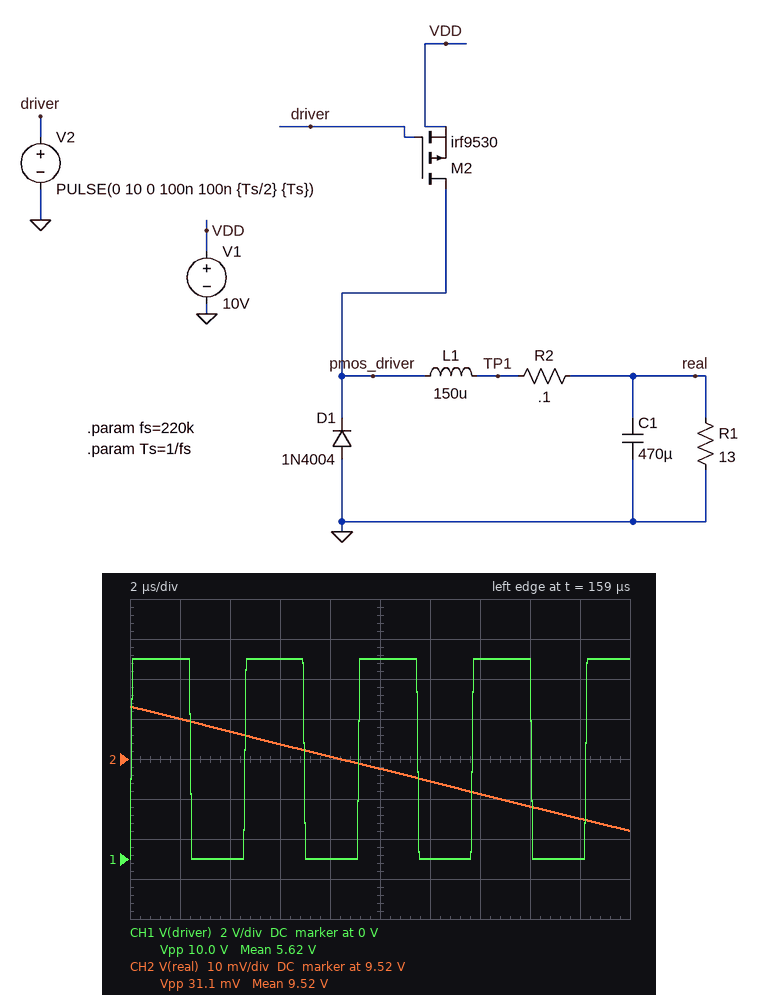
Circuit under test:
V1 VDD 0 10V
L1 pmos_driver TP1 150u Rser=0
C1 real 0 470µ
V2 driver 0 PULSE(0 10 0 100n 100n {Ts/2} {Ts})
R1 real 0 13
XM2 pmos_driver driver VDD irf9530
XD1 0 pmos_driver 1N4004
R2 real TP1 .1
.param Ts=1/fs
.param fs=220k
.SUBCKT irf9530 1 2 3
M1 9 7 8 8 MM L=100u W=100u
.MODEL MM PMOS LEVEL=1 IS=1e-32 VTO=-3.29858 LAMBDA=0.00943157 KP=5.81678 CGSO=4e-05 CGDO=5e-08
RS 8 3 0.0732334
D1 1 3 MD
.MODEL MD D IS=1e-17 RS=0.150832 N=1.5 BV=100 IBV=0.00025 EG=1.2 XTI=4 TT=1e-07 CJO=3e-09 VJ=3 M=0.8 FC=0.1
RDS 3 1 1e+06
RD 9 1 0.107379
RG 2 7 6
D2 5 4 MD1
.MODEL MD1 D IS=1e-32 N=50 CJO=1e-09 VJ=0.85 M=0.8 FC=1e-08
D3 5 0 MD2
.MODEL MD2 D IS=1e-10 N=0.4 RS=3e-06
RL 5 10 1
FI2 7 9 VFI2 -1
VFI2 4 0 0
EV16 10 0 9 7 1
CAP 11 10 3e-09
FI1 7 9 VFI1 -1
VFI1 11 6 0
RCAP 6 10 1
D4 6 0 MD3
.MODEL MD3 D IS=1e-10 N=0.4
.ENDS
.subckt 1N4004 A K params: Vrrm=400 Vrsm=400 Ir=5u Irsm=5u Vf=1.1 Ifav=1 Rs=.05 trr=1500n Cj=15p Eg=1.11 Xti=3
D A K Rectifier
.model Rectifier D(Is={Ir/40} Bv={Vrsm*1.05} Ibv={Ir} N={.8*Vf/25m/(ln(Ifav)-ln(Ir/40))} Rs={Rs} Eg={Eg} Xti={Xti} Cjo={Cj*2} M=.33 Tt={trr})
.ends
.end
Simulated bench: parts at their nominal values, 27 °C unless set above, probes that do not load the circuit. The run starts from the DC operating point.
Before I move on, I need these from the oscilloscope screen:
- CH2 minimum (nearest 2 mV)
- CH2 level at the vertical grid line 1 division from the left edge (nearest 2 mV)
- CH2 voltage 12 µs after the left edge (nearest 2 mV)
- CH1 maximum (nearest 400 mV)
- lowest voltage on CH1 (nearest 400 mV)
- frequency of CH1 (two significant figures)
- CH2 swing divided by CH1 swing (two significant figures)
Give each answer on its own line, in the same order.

9.502 V
9.530 V
9.514 V
10.0 V
0 V
220 kHz
0.0031
